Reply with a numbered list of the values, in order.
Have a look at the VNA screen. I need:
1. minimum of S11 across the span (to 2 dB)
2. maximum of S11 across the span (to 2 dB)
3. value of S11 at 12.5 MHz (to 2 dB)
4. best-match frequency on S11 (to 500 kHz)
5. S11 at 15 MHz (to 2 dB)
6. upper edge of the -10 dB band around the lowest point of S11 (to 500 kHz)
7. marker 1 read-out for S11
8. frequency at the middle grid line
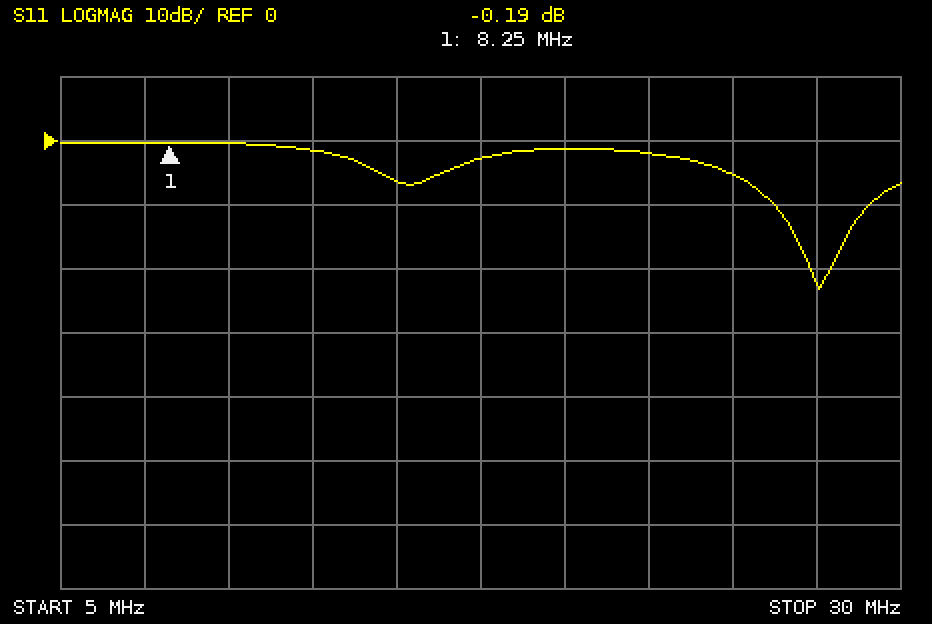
1. -24 dB
2. 0 dB
3. -2 dB
4. 27.5 MHz
5. -6 dB
6. 29.0 MHz
7. -0.19 dB
8. 17.5 MHz
